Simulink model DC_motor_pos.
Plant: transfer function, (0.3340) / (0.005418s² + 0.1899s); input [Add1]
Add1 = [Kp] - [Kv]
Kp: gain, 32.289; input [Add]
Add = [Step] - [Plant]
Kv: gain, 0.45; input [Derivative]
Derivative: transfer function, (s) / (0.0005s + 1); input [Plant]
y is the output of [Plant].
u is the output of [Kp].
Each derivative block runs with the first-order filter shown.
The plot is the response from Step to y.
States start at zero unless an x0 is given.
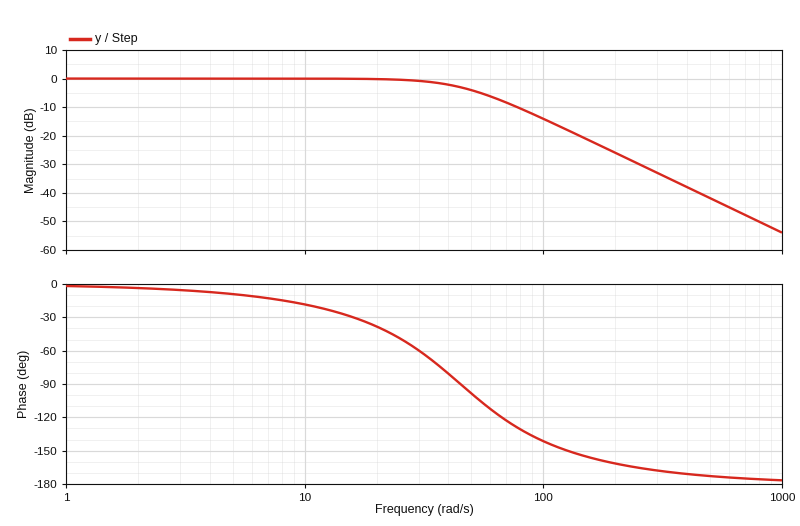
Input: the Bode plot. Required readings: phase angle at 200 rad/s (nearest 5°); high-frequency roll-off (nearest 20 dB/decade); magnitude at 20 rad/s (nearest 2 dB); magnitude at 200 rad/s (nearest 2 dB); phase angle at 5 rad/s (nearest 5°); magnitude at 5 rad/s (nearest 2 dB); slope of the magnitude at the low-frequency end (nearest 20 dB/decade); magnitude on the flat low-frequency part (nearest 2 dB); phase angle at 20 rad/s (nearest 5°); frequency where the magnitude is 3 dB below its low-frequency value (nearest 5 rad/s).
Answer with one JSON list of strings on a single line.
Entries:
["-160°", "-40 dB/decade", "0 dB", "-26 dB", "-10°", "0 dB", "0 dB/decade", "0 dB", "-40°", "45 rad/s"]
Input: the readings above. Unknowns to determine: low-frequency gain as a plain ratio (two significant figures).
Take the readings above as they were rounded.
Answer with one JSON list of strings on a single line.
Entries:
["1.0"]
